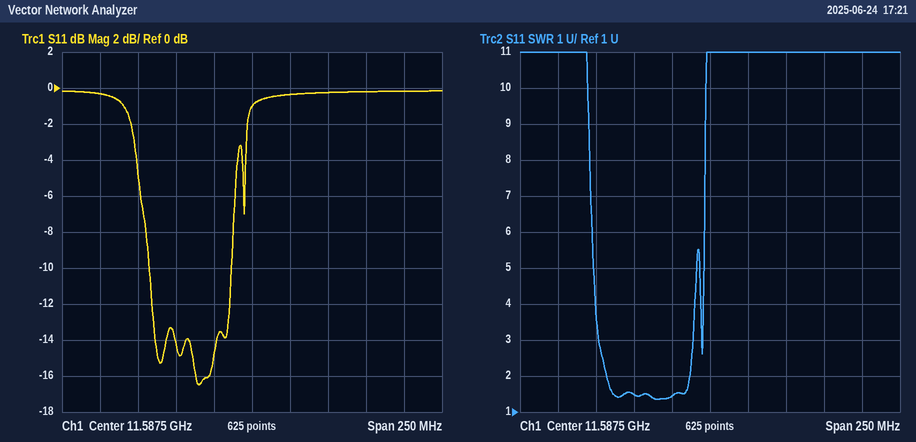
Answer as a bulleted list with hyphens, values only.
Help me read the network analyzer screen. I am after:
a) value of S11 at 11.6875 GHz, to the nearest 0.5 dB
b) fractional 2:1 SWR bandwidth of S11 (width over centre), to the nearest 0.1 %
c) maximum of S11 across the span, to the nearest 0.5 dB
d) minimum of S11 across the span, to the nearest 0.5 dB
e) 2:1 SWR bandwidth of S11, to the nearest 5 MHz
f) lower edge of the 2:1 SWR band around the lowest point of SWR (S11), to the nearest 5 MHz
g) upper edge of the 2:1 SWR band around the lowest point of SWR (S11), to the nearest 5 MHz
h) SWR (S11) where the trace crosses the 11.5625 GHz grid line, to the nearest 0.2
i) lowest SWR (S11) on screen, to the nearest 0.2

- 0.0 dB
- 0.5 %
- 0.0 dB
- -16.5 dB
- 55 MHz
- 11.520 GHz
- 11.575 GHz
- 1.4
- 1.4
